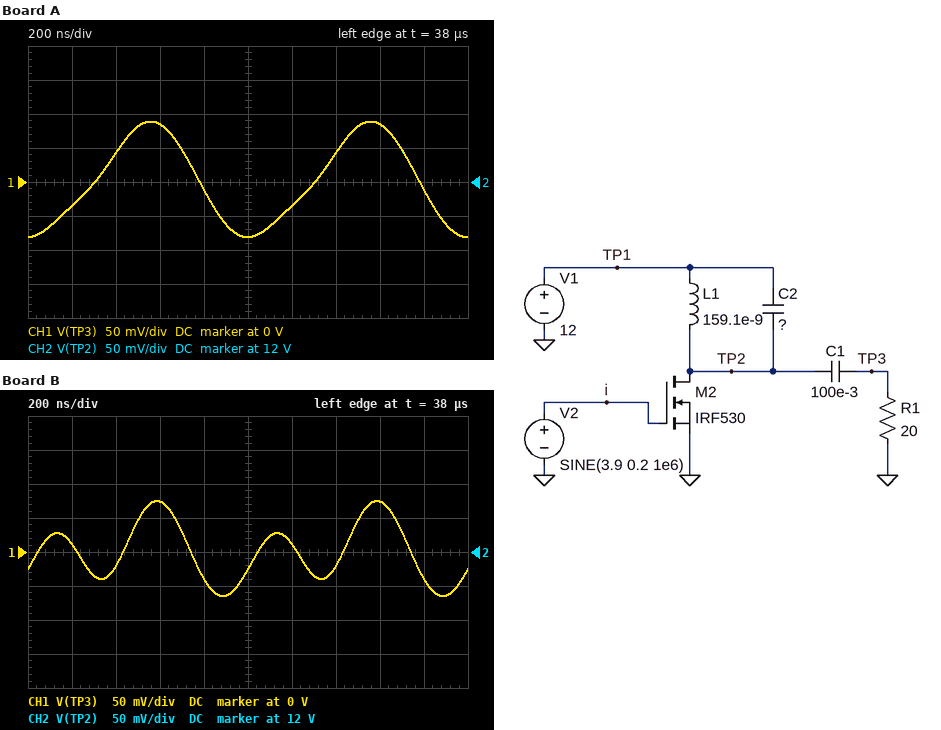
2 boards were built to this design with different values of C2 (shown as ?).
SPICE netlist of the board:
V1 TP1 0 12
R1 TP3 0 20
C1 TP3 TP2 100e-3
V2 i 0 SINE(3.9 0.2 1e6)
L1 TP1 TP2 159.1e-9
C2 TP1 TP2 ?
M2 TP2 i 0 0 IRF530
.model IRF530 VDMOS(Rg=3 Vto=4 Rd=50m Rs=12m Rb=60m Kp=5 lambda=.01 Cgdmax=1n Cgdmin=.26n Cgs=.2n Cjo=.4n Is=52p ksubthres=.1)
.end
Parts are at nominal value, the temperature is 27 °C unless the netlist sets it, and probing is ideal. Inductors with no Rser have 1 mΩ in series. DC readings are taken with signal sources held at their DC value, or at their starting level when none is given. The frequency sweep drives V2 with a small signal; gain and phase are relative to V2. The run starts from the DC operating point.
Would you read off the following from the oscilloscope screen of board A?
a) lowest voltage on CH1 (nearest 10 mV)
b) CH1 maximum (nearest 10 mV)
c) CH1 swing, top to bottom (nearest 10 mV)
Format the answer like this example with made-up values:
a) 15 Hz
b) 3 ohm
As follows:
a) -80 mV
b) 90 mV
c) 170 mV
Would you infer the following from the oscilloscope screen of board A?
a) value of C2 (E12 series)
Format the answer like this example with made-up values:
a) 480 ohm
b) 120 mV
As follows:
a) 120 nF
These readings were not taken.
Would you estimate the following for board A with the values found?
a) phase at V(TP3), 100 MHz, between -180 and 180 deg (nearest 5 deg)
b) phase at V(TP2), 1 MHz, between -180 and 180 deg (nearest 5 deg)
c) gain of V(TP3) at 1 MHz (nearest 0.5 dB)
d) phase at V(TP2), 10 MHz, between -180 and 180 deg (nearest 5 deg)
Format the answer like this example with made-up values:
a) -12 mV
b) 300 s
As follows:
a) -30 deg
b) -105 deg
c) -14.5 dB
d) 65 deg
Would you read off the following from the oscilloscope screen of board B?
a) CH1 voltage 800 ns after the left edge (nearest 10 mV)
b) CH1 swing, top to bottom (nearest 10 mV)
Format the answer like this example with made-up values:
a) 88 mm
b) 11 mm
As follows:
a) -40 mV
b) 140 mV
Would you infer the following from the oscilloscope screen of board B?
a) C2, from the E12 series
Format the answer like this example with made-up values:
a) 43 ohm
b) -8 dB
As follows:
a) 56 nF
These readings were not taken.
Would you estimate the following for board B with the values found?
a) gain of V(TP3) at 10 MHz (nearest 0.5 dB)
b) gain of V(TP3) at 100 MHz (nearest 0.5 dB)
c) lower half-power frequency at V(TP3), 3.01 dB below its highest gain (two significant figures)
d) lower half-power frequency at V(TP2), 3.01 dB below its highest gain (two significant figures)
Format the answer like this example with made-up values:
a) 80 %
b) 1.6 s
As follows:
a) -36.5 dB
b) -48.0 dB
c) 1.6 MHz
d) 1.6 MHz
